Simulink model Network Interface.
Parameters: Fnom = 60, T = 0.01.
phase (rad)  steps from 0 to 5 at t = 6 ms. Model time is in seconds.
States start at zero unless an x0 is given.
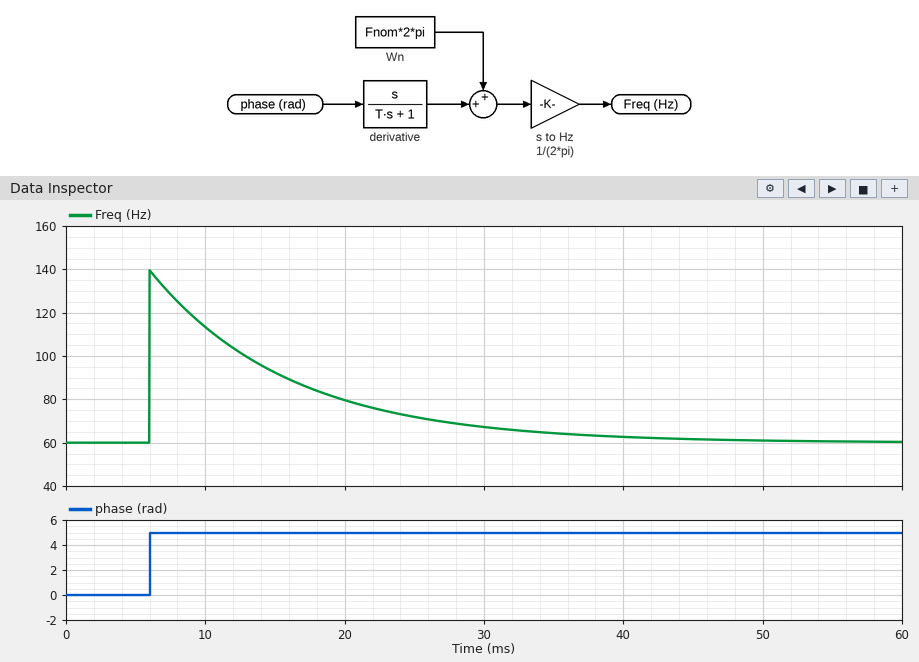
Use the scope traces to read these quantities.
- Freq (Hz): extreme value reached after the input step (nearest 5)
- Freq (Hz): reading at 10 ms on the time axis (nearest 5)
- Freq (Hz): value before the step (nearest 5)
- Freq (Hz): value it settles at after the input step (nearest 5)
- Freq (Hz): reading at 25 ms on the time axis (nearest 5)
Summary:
140
115
60
60
70
